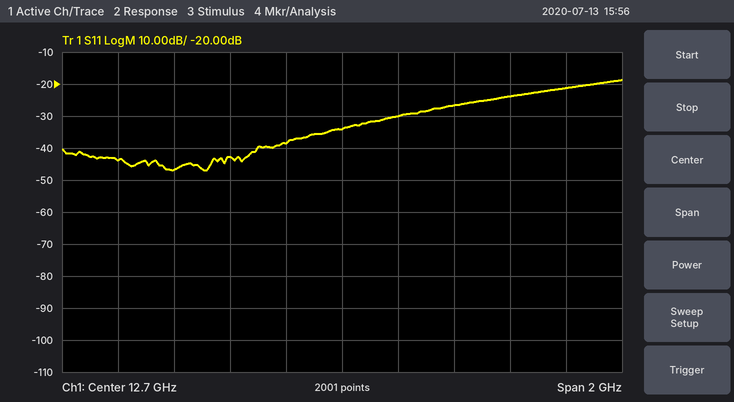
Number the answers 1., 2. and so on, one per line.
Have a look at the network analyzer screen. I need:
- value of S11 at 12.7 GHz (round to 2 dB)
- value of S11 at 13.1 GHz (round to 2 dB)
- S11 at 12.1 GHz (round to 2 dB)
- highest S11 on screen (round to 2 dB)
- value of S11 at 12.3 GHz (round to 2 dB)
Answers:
1. -34 dB
2. -26 dB
3. -46 dB
4. -18 dB
5. -42 dB
